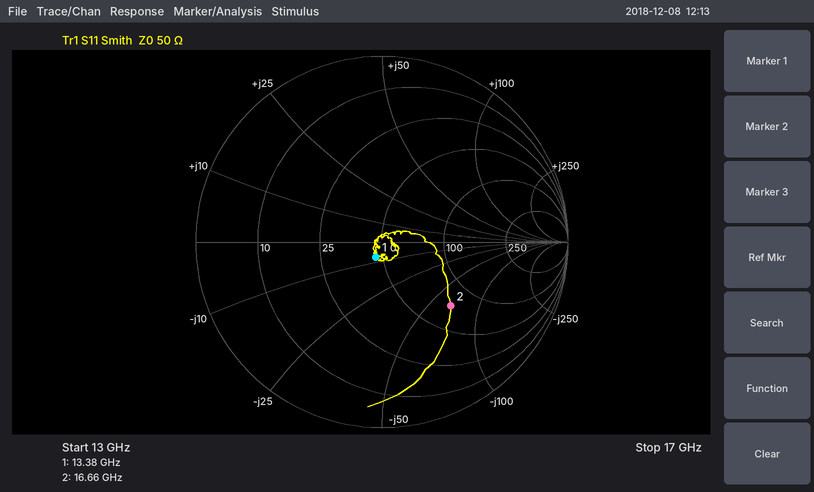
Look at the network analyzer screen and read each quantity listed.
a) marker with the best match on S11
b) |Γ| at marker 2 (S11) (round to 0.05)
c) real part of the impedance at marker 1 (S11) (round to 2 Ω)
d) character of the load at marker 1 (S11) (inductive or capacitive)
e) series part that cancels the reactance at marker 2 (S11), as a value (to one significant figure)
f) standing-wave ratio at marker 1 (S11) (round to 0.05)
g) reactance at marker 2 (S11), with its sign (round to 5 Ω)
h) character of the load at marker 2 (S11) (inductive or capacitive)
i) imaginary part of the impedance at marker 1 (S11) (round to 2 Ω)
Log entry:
marker 1
0.50
46 Ω
capacitive
600 pH
1.20
-65 Ω
capacitive
-8 Ω
